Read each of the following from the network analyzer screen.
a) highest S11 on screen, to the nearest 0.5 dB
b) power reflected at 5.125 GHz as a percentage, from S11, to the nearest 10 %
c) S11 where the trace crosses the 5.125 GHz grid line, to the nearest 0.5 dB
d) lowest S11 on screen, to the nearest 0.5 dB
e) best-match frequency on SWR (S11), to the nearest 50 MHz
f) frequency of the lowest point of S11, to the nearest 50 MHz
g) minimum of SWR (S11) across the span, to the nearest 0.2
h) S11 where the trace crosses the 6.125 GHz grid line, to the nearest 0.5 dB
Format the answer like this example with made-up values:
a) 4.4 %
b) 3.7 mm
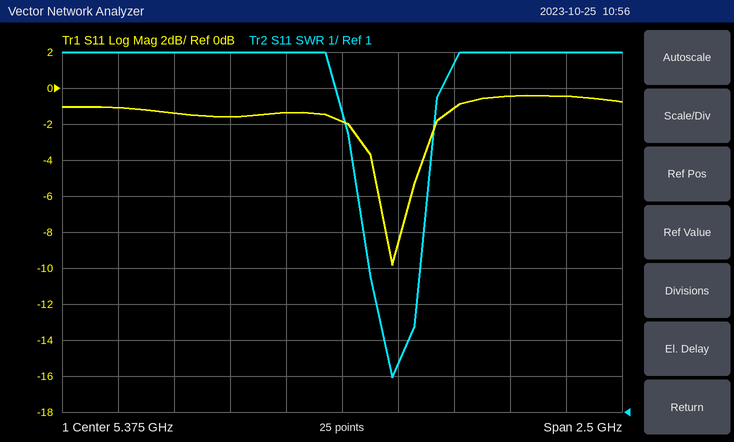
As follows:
a) -0.5 dB
b) 70 %
c) -1.5 dB
d) -10.0 dB
e) 5.60 GHz
f) 5.60 GHz
g) 2.0
h) -0.5 dB
